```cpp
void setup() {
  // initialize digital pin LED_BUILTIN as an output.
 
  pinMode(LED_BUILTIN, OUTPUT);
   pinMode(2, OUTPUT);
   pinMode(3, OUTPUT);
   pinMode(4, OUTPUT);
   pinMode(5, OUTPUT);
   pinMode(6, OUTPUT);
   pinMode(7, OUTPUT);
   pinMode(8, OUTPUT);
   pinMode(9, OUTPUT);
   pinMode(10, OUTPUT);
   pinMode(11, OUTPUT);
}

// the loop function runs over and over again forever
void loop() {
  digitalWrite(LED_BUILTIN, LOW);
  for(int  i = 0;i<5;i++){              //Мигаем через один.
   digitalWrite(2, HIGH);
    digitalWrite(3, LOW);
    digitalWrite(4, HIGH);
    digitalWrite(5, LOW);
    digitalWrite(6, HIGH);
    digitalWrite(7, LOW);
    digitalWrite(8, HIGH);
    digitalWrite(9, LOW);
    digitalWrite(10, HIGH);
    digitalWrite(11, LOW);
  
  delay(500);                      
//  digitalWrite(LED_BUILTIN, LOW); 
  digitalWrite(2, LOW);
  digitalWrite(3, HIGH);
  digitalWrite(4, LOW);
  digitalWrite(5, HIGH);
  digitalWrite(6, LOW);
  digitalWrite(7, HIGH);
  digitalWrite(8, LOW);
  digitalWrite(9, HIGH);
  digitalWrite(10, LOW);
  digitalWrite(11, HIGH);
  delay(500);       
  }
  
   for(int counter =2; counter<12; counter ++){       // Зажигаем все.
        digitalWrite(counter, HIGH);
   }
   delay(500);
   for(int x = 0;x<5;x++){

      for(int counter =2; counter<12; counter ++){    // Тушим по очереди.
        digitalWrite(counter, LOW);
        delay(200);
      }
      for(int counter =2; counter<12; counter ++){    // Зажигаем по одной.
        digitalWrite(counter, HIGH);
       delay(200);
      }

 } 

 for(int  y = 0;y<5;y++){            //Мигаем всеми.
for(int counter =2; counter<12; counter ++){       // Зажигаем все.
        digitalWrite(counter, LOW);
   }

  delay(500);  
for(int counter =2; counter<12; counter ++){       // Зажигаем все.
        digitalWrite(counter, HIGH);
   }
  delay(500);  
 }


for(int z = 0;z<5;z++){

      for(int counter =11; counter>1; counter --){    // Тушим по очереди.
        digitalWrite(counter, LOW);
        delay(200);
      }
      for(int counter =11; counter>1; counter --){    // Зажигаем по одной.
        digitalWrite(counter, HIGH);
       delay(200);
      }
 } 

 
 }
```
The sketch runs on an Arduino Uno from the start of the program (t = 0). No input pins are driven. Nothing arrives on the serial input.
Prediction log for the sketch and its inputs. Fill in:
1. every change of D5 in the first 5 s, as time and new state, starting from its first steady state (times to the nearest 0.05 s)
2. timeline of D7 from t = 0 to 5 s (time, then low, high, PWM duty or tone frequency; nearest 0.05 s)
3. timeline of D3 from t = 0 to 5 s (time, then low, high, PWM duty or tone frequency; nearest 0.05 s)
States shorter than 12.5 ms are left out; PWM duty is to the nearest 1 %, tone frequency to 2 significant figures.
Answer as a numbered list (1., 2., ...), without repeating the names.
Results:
1. 0 s low; 0.5 s high; 1 s low; 1.5 s high; 2 s low; 2.5 s high; 3 s low; 3.5 s high; 4 s low; 4.5 s high
2. 0 s low; 0.5 s high; 1 s low; 1.5 s high; 2 s low; 2.5 s high; 3 s low; 3.5 s high; 4 s low; 4.5 s high
3. 0 s low; 0.5 s high; 1 s low; 1.5 s high; 2 s low; 2.5 s high; 3 s low; 3.5 s high; 4 s low; 4.5 s high
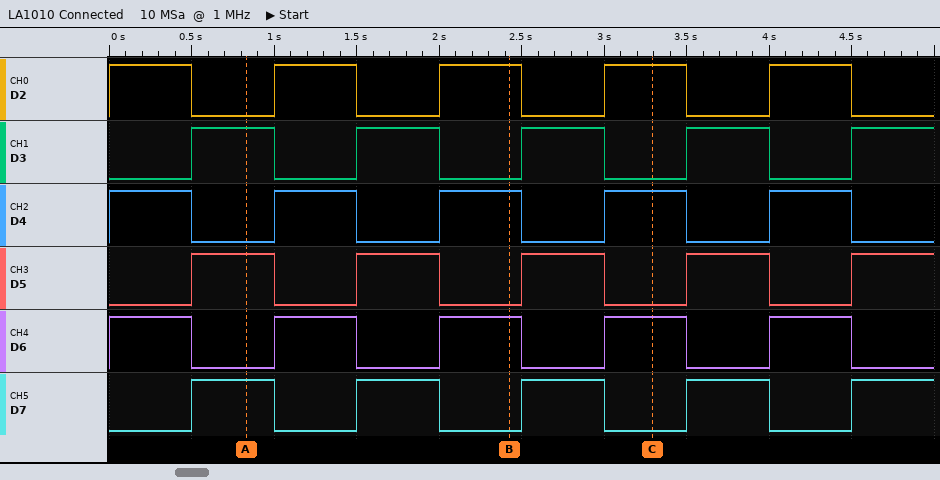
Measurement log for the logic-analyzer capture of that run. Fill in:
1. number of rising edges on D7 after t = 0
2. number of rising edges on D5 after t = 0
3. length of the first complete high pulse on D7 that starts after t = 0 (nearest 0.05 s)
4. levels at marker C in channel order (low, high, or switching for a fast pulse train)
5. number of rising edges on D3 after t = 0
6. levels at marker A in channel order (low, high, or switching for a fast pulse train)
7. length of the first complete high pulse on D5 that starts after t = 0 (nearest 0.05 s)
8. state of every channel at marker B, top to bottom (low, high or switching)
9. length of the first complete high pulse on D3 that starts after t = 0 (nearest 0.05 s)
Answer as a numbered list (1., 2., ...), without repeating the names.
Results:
1. 5
2. 5
3. 0.50 s
4. D2 high, D3 low, D4 high, D5 low, D6 high, D7 low
5. 5
6. D2 low, D3 high, D4 low, D5 high, D6 low, D7 high
7. 0.50 s
8. D2 high, D3 low, D4 high, D5 low, D6 high, D7 low
9. 0.50 s
